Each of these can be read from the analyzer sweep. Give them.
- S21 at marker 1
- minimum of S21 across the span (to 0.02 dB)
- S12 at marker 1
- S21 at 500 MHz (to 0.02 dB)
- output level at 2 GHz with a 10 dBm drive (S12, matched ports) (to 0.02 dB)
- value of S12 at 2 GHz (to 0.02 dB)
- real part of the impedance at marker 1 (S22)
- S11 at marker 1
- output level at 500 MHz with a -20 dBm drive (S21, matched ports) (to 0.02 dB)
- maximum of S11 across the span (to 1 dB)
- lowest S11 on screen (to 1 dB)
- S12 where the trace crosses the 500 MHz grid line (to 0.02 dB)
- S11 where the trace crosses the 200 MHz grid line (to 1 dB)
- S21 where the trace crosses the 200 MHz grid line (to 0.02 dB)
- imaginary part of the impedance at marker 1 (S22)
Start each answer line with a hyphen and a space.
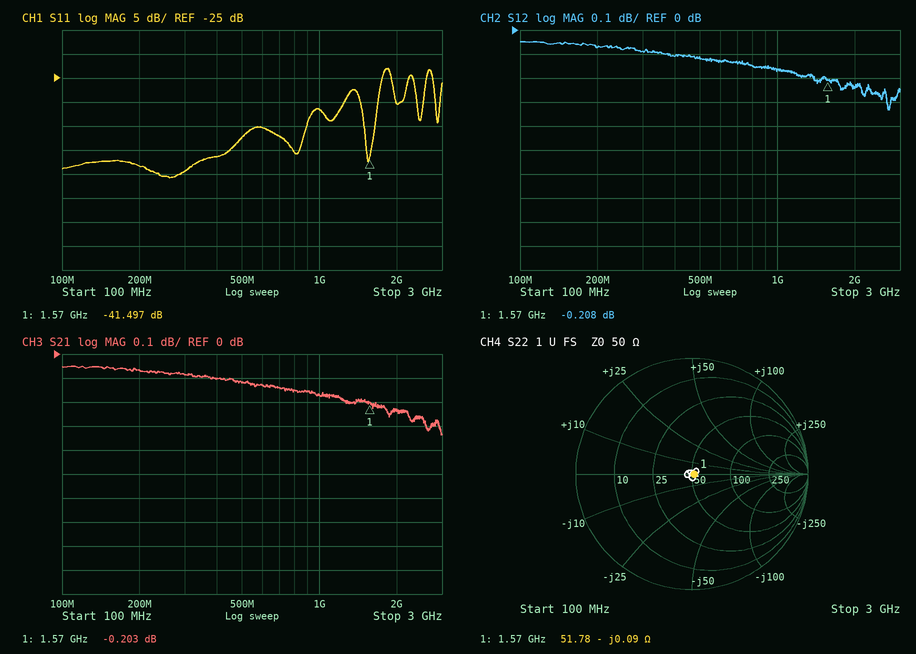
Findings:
- -0.203 dB
- -0.34 dB
- -0.208 dB
- -0.12 dB
- 9.76 dBm
- -0.24 dB
- 51.78 Ω
- -41.497 dB
- -20.12 dBm
- -23 dB
- -46 dB
- -0.12 dB
- -43 dB
- -0.06 dB
- -0.09 Ω
